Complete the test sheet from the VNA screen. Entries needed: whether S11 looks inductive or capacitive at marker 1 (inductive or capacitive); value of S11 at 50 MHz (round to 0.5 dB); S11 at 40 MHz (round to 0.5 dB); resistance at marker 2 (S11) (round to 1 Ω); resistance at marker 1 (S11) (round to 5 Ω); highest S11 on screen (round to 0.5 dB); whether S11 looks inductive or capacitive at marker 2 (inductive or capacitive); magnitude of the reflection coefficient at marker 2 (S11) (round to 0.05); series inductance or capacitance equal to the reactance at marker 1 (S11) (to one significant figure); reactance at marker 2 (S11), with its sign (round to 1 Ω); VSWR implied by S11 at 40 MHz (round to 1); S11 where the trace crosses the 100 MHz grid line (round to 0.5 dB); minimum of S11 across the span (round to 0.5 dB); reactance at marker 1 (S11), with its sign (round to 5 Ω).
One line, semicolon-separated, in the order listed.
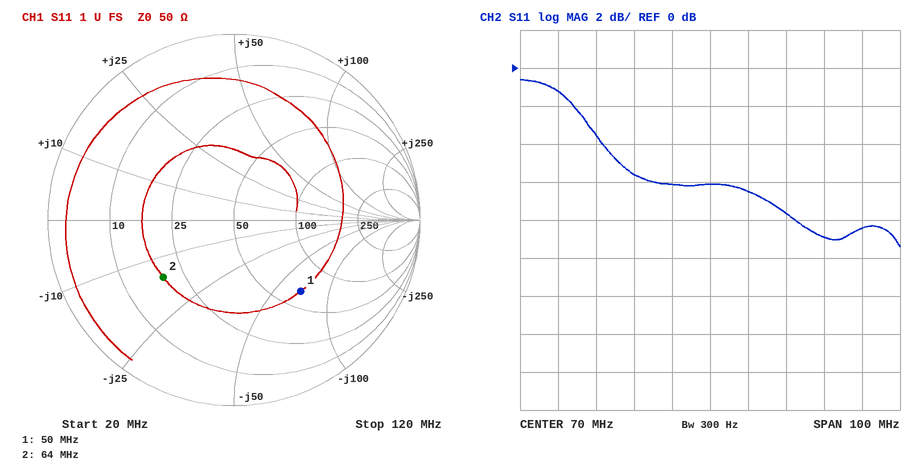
capacitive; -5.5 dB; -3.5 dB; 19 Ω; 65 Ω; -0.5 dB; capacitive; 0.50; 50 pF; -15 Ω; 5; -9.0 dB; -9.5 dB; -70 Ω
